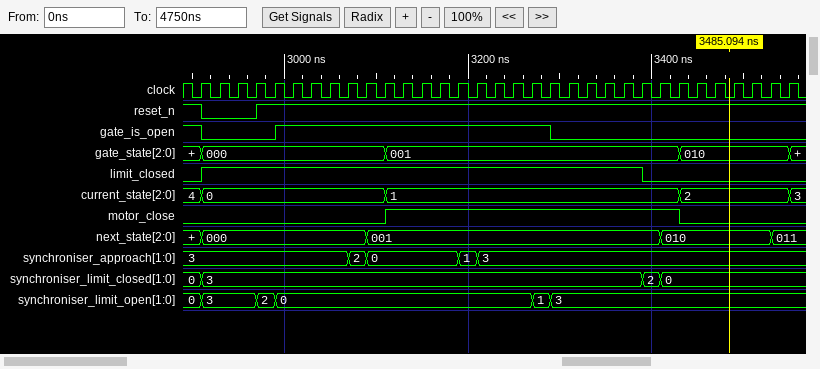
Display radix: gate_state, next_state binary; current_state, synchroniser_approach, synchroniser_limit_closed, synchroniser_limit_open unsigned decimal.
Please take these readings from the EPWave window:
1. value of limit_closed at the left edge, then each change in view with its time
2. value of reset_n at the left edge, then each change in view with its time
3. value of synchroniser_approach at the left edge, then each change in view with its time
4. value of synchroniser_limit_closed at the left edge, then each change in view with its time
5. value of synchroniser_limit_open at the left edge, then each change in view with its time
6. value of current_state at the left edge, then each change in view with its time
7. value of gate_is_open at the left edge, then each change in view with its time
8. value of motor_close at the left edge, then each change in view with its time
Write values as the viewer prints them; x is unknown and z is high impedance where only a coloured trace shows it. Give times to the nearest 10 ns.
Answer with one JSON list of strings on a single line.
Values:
["0, 1 at 2910 ns, 0 at 3390 ns", "1, 0 at 2910 ns, 1 at 2970 ns", "3, 2 at 3070 ns, 0 at 3090 ns, 1 at 3190 ns, 3 at 3210 ns", "0, 3 at 2910 ns, 2 at 3390 ns, 0 at 3410 ns", "0, 3 at 2910 ns, 2 at 2970 ns, 0 at 2990 ns, 1 at 3270 ns, 3 at 3290 ns", "4, 0 at 2910 ns, 1 at 3110 ns, 2 at 3430 ns, 3 at 3550 ns", "1, 0 at 2910 ns, 1 at 2990 ns, 0 at 3290 ns", "0, 1 at 3110 ns, 0 at 3430 ns"]
